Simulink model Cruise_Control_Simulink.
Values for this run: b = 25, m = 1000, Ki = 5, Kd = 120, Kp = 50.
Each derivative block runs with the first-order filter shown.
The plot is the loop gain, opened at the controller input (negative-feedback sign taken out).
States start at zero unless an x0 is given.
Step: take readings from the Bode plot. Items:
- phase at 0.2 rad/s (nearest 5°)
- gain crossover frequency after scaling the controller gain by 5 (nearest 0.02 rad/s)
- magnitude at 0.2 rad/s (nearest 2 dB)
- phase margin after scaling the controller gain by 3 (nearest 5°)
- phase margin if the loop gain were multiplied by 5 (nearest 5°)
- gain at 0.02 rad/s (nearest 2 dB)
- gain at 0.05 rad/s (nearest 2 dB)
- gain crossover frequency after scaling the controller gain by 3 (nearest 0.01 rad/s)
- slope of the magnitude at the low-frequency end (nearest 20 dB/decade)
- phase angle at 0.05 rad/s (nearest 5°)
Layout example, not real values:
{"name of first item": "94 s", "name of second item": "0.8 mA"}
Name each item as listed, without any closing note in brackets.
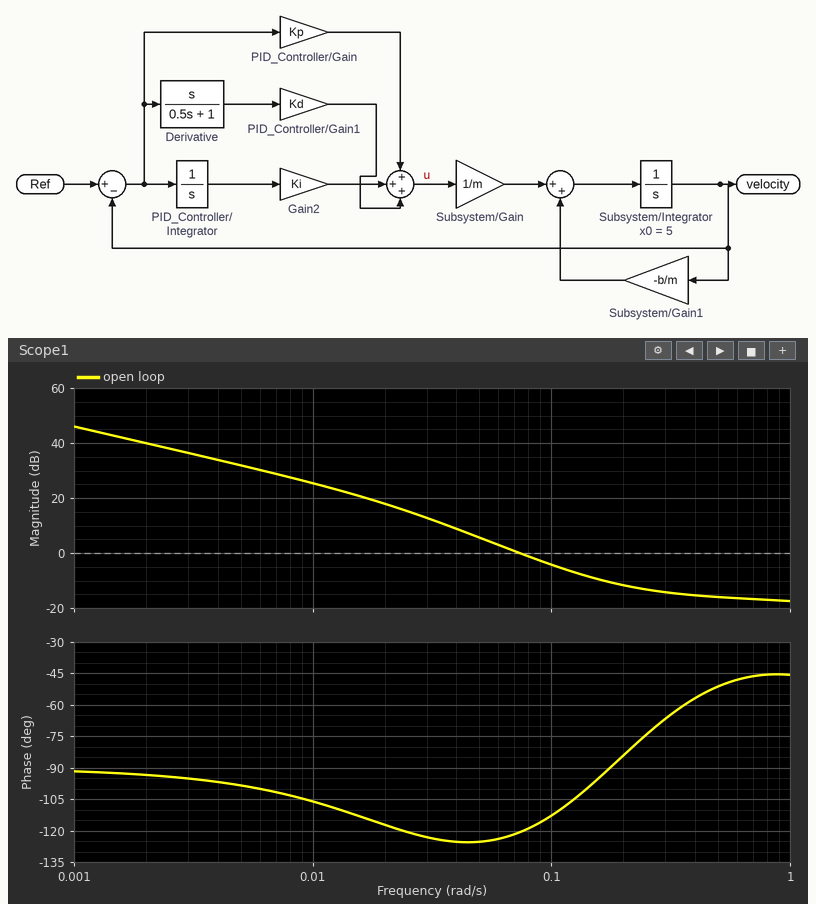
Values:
{"phase at 0.2 rad/s": "-85°", "gain crossover frequency after scaling the controller gain by 5": "0.28 rad/s", "magnitude at 0.2 rad/s": "-12 dB", "phase margin after scaling the controller gain by 3": "85°", "phase margin if the loop gain were multiplied by 5": "110°", "gain at 0.02 rad/s": "18 dB", "gain at 0.05 rad/s": "6 dB", "gain crossover frequency after scaling the controller gain by 3": "0.16 rad/s", "slope of the magnitude at the low-frequency end": "-20 dB/decade", "phase angle at 0.05 rad/s": "-125°"}
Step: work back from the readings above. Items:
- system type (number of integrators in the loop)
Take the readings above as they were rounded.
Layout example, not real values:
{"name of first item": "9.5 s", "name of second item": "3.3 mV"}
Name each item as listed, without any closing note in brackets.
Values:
{"system type": "1"}
